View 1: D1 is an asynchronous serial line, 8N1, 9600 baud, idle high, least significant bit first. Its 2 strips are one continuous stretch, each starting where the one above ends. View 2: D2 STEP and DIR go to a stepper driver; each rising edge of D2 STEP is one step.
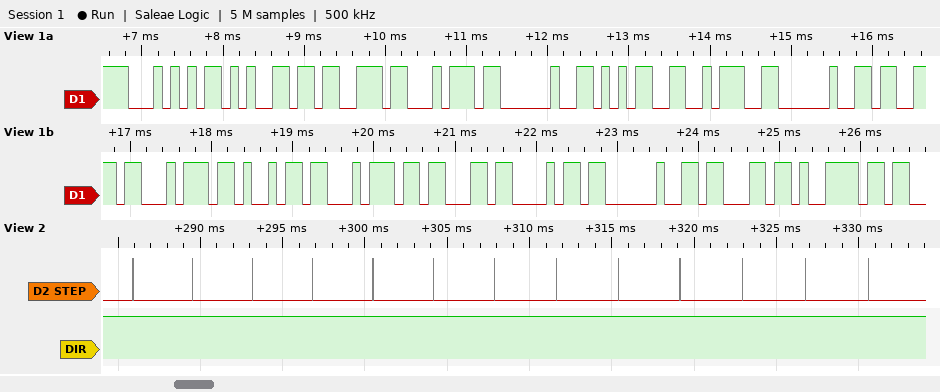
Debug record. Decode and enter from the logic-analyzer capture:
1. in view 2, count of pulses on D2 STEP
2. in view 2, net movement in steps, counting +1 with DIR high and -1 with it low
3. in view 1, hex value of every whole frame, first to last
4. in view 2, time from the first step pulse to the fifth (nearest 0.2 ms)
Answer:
13
+13
0x54 0x65 0x73 0x74 0x20 0x35 0x3A 0x20 0x73 0x74 0x69 0x74 0x63 0x68 0x20 0x63 0x79
14.6 ms
